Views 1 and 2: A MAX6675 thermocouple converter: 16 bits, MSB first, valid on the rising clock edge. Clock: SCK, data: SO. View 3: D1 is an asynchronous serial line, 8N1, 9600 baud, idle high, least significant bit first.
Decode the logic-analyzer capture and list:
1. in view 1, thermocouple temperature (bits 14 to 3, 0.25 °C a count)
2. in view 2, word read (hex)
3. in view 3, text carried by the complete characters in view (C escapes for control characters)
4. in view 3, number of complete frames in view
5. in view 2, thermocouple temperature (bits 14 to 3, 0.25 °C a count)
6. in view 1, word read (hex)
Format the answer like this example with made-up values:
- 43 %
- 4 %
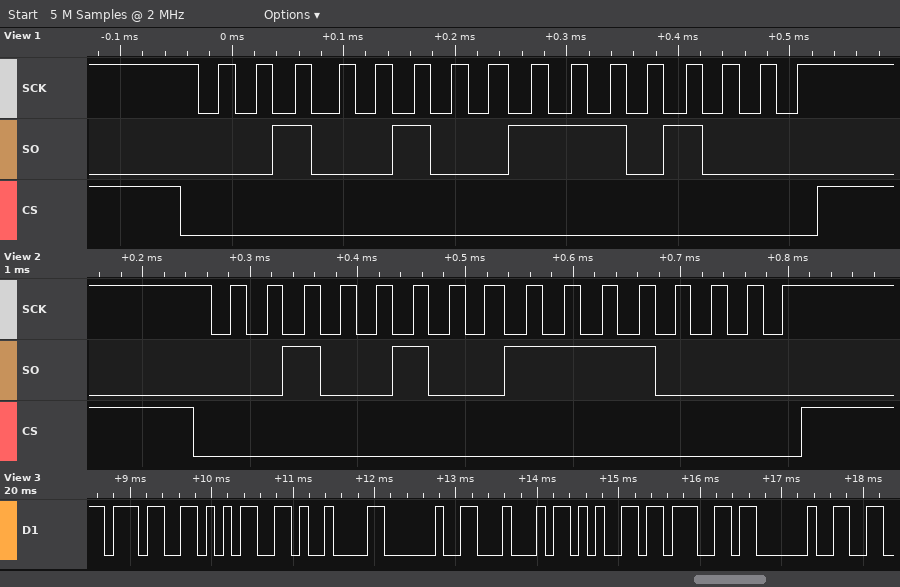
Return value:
- 295.25 °C
- 0x24F0
- "75\t Deg "
- 8
- 295.50 °C
- 0x24E8
